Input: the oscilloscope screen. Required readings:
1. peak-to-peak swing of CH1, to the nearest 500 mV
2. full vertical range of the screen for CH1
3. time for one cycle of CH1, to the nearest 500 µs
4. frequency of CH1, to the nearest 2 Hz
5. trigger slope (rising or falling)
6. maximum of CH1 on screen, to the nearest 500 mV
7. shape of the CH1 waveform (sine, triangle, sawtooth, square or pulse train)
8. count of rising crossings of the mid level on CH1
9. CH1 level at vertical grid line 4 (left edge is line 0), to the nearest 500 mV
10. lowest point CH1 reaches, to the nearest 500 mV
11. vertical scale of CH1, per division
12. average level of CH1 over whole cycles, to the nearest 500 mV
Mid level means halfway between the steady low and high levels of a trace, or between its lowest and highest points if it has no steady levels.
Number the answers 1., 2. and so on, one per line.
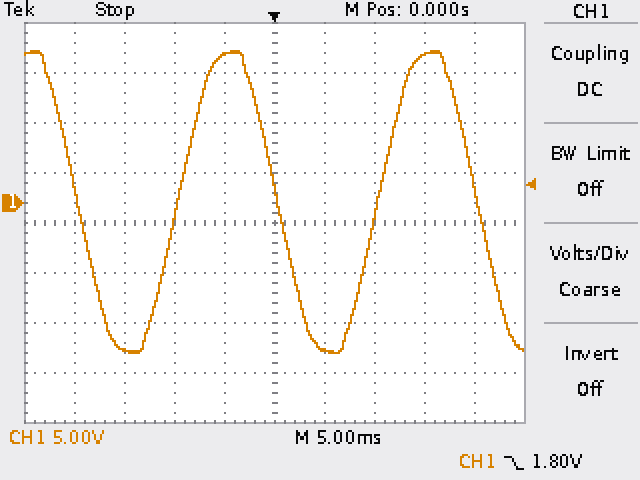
1. 30.0 V
2. 40 V
3. 20.0 ms
4. 50 Hz
5. falling
6. 15.0 V
7. sine
8. 2
9. 15.0 V
10. -15.0 V
11. 5 V
12. 0.0 V
